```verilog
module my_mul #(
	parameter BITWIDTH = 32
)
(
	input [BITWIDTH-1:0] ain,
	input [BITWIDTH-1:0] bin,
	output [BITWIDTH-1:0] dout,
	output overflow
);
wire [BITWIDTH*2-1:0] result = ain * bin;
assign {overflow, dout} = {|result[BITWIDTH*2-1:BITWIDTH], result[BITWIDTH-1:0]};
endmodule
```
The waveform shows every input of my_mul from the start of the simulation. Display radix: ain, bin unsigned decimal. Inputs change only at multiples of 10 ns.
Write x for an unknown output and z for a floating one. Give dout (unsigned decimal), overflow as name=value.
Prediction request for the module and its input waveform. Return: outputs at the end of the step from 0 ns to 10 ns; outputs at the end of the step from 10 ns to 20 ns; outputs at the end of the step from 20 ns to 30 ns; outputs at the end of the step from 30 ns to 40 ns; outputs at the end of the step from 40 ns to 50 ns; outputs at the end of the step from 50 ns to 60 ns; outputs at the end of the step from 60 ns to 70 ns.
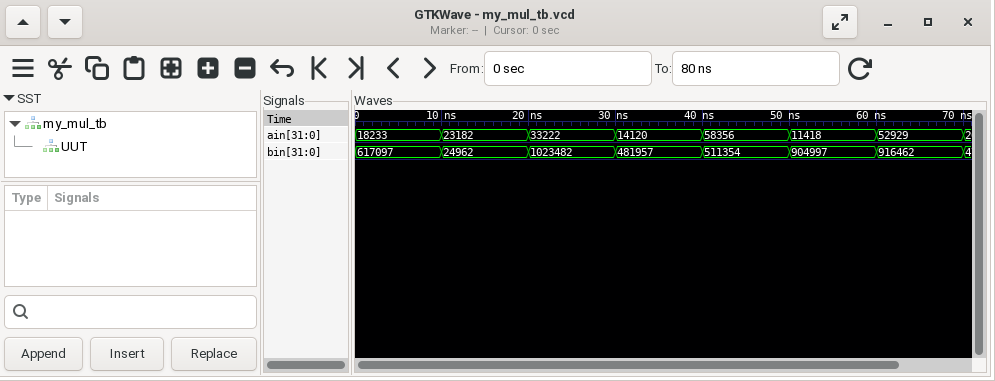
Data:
dout=2661595009, overflow=1
dout=578669084, overflow=0
dout=3937347932, overflow=1
dout=2510265544, overflow=1
dout=4070770248, overflow=1
dout=1743321154, overflow=1
dout=1262776942, overflow=1
